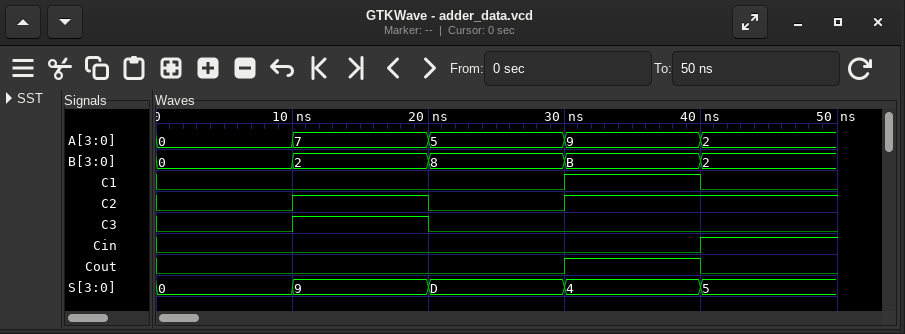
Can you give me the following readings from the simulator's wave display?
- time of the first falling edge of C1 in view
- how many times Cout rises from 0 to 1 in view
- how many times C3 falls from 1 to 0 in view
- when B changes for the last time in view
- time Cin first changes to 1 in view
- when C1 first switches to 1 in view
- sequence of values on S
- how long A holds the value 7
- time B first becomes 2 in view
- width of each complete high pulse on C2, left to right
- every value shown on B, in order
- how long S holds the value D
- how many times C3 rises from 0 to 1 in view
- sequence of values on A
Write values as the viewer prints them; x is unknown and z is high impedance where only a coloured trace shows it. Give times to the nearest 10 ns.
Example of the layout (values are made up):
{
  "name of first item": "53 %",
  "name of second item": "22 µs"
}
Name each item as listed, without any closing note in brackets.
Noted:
{
  "time of the first falling edge of C1 in view": "40 ns",
  "how many times Cout rises from 0 to 1 in view": "1",
  "how many times C3 falls from 1 to 0 in view": "1",
  "when B changes for the last time in view": "40 ns",
  "time Cin first changes to 1 in view": "40 ns",
  "when C1 first switches to 1 in view": "30 ns",
  "sequence of values on S": "0, 9, D, 4, 5",
  "how long A holds the value 7": "10 ns",
  "time B first becomes 2 in view": "10 ns",
  "width of each complete high pulse on C2, left to right": "10 ns",
  "every value shown on B, in order": "0, 2, 8, B, 2",
  "how long S holds the value D": "10 ns",
  "how many times C3 rises from 0 to 1 in view": "1",
  "sequence of values on A": "0, 7, 5, 9, 2"
}
